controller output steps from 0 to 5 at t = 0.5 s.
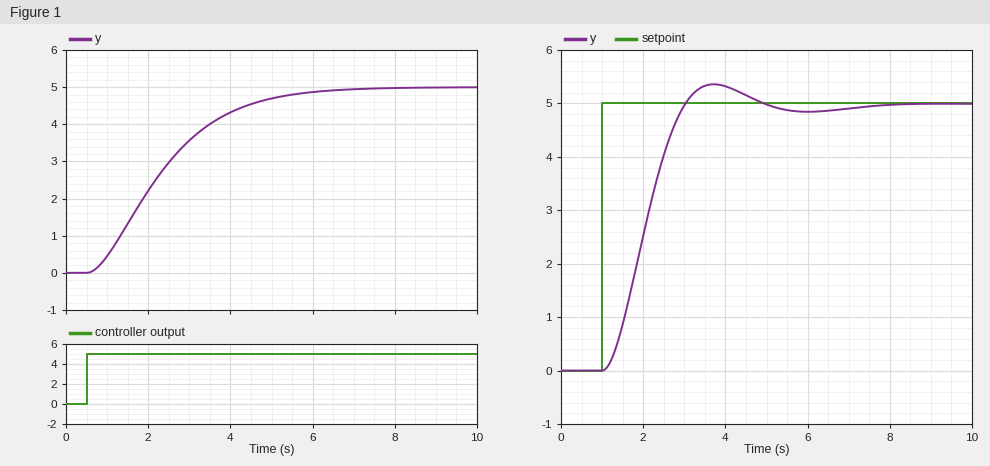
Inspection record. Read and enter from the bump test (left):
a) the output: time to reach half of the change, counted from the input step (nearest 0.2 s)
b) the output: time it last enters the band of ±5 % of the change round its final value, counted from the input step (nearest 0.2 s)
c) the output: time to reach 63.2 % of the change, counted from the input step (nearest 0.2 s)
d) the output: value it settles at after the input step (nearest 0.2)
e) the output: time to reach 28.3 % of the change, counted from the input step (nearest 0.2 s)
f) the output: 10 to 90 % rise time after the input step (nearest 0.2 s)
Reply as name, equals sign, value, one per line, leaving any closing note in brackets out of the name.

the output: time to reach half of the change, counted from the input step = 1.6 s
the output: time it last enters the band of ±5 % of the change round its final value, counted from the input step = 4.8 s
the output: time to reach 63.2 % of the change, counted from the input step = 2.2 s
the output: value it settles at after the input step = 5.0
the output: time to reach 28.3 % of the change, counted from the input step = 1.0 s
the output: 10 to 90 % rise time after the input step = 3.4 s
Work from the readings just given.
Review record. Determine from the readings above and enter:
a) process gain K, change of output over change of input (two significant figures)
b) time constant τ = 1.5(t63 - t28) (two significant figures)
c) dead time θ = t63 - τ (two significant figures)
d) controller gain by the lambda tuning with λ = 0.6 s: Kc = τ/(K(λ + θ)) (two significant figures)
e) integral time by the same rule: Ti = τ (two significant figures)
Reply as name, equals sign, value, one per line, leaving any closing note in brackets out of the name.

process gain K, change of output over change of input = 1.0
time constant τ = 1.5(t63 - t28) = 1.8 s
dead time θ = t63 - τ = 0.40 s
controller gain by the lambda tuning with λ = 0.6 s: Kc = τ/(K(λ + θ)) = 1.8
integral time by the same rule: Ti = τ = 1.8 s
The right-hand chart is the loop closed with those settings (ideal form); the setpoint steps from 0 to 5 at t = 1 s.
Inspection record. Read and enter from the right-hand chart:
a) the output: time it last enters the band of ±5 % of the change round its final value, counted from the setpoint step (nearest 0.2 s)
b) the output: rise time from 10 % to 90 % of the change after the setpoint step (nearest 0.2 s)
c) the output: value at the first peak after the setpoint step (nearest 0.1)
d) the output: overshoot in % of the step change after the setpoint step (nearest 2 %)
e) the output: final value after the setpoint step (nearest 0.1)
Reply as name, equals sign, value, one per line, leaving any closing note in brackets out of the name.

the output: time it last enters the band of ±5 % of the change round its final value, counted from the setpoint step = 3.2 s
the output: rise time from 10 % to 90 % of the change after the setpoint step = 1.4 s
the output: value at the first peak after the setpoint step = 5.4
the output: overshoot in % of the step change after the setpoint step = 8 %
the output: final value after the setpoint step = 5.0
